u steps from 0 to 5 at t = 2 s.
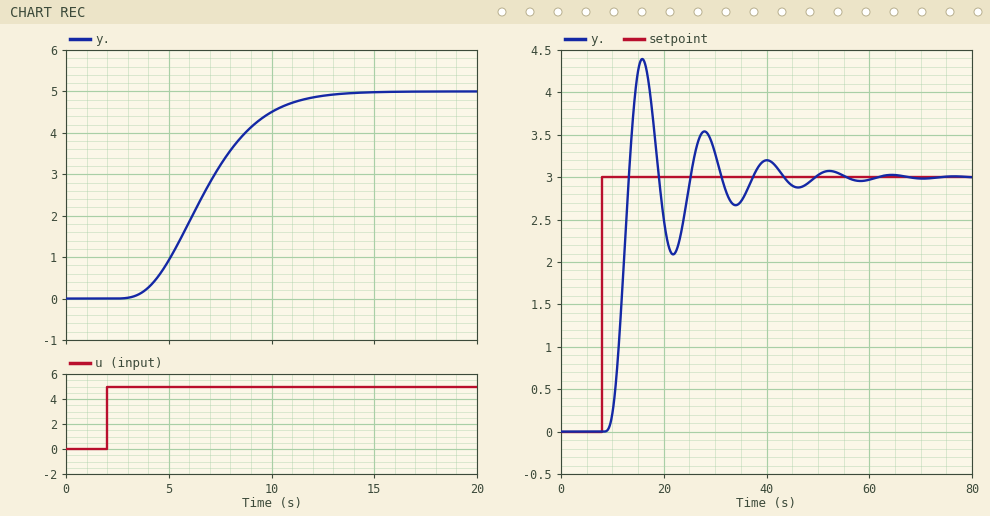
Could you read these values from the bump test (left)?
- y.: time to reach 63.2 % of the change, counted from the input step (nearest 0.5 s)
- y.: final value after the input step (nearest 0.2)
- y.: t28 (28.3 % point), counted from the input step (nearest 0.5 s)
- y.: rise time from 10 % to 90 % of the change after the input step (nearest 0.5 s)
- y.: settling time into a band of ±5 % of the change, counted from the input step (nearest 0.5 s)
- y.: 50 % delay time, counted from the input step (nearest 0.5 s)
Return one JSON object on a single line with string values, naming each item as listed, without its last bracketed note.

{"y.: time to reach 63.2 % of the change, counted from the input step": "5.5 s", "y.: final value after the input step": "5.0", "y.: t28 (28.3 % point), counted from the input step": "3.5 s", "y.: rise time from 10 % to 90 % of the change after the input step": "5.5 s", "y.: settling time into a band of ±5 % of the change, counted from the input step": "9.0 s", "y.: 50 % delay time, counted from the input step": "4.5 s"}
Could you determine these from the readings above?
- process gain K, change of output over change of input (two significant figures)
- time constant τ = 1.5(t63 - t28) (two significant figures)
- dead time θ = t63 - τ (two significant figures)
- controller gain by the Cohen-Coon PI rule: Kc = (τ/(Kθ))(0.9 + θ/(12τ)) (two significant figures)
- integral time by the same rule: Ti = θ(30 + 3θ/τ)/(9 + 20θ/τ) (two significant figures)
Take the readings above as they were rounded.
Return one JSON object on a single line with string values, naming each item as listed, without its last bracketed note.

{"process gain K, change of output over change of input": "1.0", "time constant τ = 1.5(t63 - t28)": "3.0 s", "dead time θ = t63 - τ": "2.5 s", "controller gain by the Cohen-Coon PI rule: Kc = (τ/(Kθ))(0.9 + θ/(12τ))": "1.2", "integral time by the same rule: Ti = θ(30 + 3θ/τ)/(9 + 20θ/τ)": "3.2 s"}
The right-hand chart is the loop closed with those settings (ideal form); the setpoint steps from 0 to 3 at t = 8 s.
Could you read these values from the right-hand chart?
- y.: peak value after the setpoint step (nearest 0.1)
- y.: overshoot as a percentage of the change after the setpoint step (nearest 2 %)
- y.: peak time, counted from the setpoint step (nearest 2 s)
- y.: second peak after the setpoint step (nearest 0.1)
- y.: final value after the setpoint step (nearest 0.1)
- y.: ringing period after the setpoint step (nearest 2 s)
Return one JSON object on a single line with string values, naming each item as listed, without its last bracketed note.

{"y.: peak value after the setpoint step": "4.4", "y.: overshoot as a percentage of the change after the setpoint step": "46 %", "y.: peak time, counted from the setpoint step": "8 s", "y.: second peak after the setpoint step": "3.5", "y.: final value after the setpoint step": "3.0", "y.: ringing period after the setpoint step": "12 s"}
